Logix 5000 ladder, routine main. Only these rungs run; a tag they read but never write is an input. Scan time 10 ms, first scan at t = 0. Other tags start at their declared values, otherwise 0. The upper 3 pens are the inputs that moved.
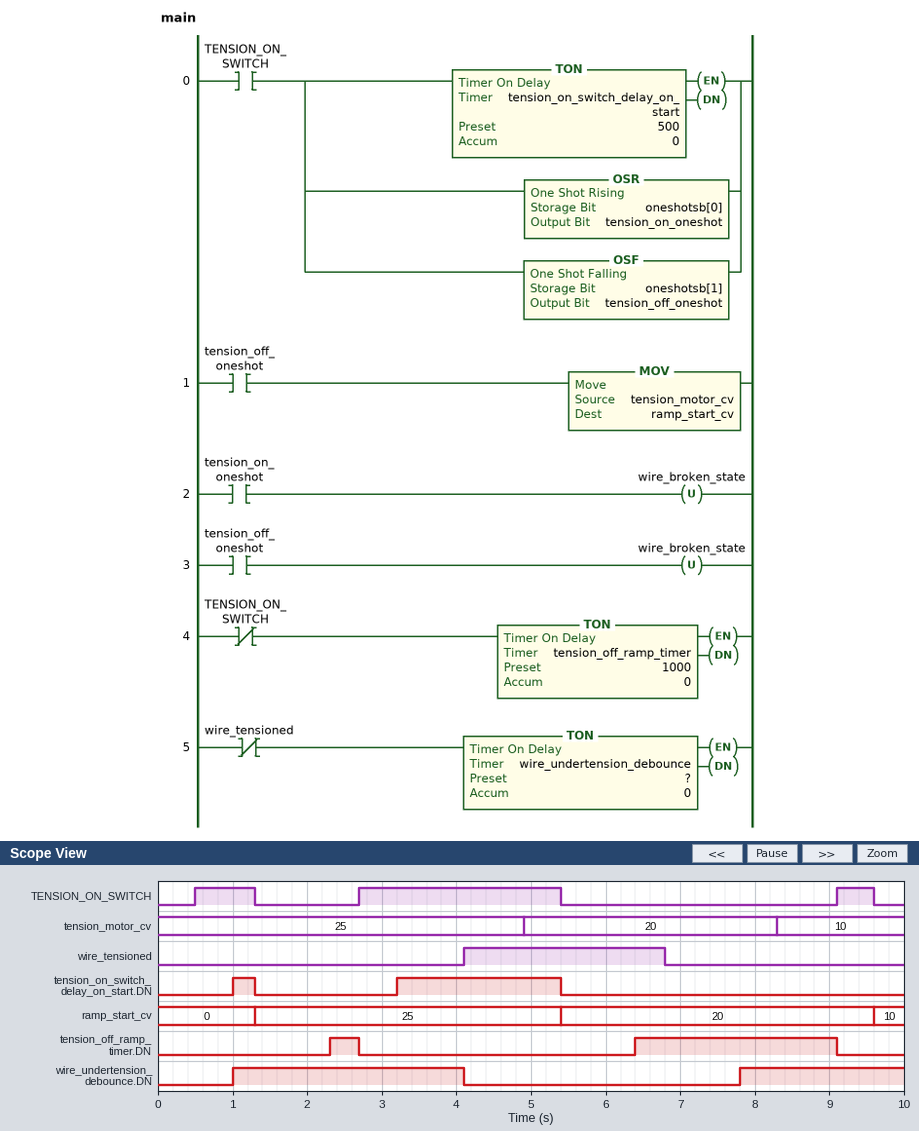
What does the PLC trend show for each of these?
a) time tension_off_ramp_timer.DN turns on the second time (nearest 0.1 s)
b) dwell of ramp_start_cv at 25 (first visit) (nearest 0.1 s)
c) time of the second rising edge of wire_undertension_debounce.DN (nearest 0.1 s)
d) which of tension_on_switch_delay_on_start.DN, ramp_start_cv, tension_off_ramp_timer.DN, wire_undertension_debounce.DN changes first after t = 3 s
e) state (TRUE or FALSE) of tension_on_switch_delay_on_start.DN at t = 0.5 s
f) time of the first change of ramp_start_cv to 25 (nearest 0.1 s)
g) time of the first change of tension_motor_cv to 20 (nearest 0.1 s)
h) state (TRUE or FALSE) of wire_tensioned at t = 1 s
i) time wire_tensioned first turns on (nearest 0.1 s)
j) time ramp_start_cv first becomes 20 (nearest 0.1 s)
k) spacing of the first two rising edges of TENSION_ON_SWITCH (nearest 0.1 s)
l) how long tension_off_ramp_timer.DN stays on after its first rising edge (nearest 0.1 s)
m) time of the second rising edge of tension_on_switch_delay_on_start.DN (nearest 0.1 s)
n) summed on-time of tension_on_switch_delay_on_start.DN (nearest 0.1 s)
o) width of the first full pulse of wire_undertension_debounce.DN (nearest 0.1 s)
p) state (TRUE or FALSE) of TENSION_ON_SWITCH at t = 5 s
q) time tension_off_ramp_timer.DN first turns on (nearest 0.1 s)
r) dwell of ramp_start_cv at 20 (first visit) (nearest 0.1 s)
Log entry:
6.4 s
4.1 s
7.8 s
tension_on_switch_delay_on_start.DN
FALSE
1.3 s
4.9 s
FALSE
4.1 s
5.4 s
2.2 s
0.4 s
3.2 s
2.5 s
3.1 s
TRUE
2.3 s
4.2 s
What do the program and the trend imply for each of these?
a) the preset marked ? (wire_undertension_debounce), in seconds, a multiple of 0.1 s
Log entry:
1.0 s
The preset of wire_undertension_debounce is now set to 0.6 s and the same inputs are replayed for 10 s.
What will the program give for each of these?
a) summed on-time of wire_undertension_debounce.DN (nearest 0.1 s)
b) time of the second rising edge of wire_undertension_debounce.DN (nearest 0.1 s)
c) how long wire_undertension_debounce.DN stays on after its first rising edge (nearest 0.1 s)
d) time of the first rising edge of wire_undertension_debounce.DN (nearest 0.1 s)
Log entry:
6.1 s
7.4 s
3.5 s
0.6 s
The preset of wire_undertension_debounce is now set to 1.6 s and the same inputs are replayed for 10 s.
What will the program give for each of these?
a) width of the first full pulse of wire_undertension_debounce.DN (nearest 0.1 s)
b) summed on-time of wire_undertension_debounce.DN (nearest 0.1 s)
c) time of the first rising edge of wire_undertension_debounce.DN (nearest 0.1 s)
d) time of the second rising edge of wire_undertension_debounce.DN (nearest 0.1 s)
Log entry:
2.5 s
4.1 s
1.6 s
8.4 s
